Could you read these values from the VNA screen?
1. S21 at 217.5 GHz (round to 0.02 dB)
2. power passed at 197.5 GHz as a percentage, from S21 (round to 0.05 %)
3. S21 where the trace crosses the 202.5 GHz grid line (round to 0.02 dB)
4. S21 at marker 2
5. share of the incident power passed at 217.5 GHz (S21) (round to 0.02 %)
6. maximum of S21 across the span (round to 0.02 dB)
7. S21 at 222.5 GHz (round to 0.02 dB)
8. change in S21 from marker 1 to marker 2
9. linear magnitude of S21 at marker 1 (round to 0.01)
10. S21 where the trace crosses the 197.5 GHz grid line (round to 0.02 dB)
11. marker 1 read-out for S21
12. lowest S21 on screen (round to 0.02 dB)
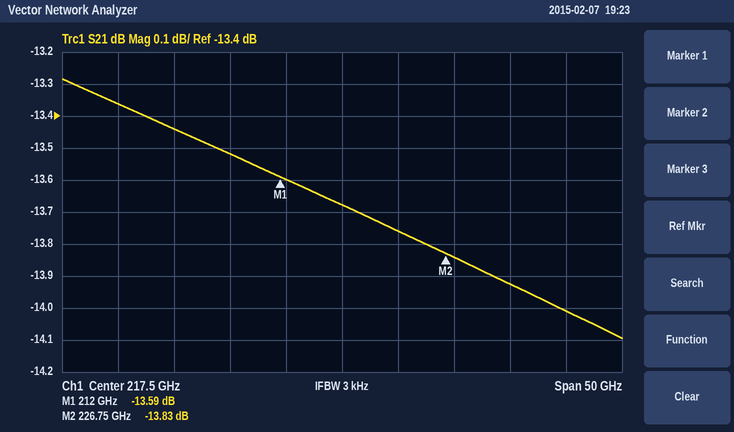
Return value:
-13.68 dB
4.60 %
-13.44 dB
-13.83 dB
4.28 %
-13.28 dB
-13.76 dB
-0.24 dB
0.21
-13.36 dB
-13.59 dB
-14.10 dB
